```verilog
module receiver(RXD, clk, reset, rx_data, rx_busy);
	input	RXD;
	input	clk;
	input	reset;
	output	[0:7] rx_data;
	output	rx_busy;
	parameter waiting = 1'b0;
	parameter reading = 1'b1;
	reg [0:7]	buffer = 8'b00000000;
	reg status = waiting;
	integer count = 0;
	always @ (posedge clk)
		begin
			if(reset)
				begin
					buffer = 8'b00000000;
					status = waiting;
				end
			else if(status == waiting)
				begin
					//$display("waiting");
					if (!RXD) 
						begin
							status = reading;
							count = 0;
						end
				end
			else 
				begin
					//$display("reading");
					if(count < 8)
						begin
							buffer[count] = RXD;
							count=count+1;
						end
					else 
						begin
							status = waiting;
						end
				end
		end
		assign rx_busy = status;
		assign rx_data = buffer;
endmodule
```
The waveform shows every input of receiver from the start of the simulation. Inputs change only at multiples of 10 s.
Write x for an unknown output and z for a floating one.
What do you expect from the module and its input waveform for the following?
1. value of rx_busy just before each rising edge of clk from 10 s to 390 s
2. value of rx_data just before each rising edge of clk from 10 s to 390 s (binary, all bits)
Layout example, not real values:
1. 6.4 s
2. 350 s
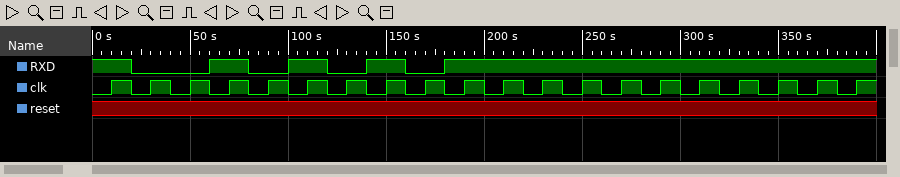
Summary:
1. 0 0 1 1 1 1 1 1 1 1 1 0 0 0 0 0 0 0 0 0
2. 00000000, 00000000, 00000000, 00000000, 01000000, 01000000, 01010000, 01010000, 01010100, 01010100, 01010101, 01010101, 01010101, 01010101, 01010101, 01010101, 01010101, 01010101, 01010101, 01010101
